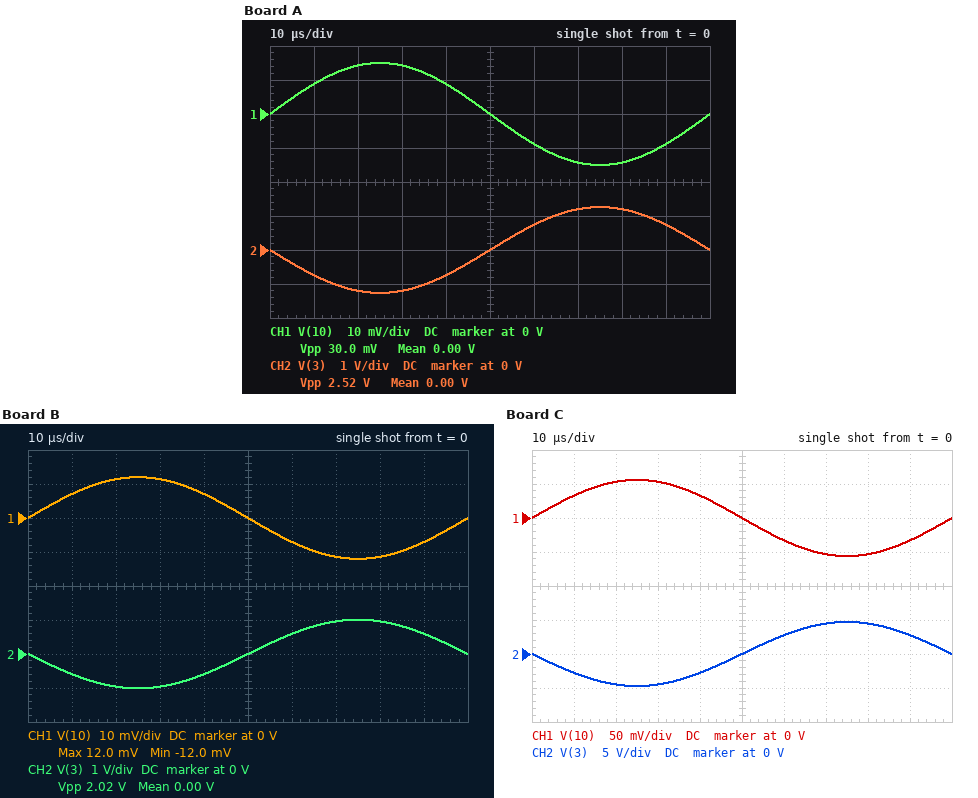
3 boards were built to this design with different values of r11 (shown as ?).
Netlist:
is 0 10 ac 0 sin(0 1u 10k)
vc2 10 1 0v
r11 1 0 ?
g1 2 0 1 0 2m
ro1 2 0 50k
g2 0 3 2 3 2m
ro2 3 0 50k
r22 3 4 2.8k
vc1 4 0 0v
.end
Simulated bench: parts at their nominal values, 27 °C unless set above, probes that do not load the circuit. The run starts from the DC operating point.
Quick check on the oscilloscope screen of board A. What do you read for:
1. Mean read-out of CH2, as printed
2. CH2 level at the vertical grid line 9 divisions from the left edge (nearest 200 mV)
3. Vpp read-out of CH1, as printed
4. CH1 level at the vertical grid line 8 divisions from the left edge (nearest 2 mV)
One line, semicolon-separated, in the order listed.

0.00 V; 800 mV; 30.0 mV; -14 mV
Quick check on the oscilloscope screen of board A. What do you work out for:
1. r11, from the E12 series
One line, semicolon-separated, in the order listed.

15 kΩ
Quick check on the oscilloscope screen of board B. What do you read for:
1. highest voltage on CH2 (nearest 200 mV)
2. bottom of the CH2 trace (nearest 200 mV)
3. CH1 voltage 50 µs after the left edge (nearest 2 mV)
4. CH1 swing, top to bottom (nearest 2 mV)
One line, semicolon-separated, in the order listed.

1.0 V; -1.0 V; 0 V; 24 mV
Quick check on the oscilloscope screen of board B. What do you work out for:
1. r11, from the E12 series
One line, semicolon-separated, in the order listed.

12 kΩ
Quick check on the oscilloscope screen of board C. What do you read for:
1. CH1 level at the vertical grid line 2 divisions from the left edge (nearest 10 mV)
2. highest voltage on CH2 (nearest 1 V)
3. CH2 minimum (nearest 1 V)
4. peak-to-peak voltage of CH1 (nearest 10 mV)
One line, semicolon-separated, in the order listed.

50 mV; 5 V; -5 V; 110 mV
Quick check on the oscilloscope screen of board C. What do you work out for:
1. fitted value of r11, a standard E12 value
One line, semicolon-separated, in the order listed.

56 kΩ
